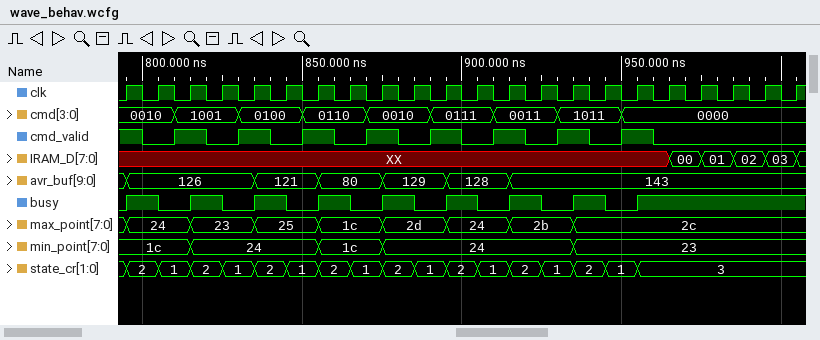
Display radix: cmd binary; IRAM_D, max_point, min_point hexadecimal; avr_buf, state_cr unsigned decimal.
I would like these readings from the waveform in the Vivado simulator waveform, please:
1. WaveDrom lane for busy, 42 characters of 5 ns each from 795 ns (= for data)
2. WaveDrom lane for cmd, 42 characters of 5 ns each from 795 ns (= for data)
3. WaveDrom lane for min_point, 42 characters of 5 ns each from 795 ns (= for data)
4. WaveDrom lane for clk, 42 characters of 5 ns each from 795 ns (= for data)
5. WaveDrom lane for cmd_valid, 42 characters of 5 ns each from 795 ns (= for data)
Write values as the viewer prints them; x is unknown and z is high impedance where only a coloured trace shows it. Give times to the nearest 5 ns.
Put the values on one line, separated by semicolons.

{name: 'busy', wave: '1.0.1.0.1.0.1.0.1.0.1.0.1.0.1.0.1.........'}; {name: 'cmd', wave: '=..=...=...=...=...=...=...=...=..........', data: '0010 1001 0100 0110 0010 0111 0011 1011 0000'}; {name: 'min_point', wave: '=...=.......=...=...........=.............', data: '1c 24 1c 24 23'}; {name: 'clk', wave: '101010101010101010101010101010101010101010'}; {name: 'cmd_valid', wave: '10.1.0.1.0.1.0.1.0.1.0.1.0.1.0.1.0........'}
